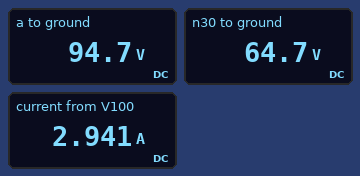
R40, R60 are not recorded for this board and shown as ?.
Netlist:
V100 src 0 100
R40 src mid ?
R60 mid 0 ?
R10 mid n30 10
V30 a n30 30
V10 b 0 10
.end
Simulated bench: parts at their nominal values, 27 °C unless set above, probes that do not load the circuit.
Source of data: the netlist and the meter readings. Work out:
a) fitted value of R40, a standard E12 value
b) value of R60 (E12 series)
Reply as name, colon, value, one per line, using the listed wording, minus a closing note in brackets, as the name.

fitted value of R40, a standard E12 value: 12 Ω
value of R60: 22 Ω
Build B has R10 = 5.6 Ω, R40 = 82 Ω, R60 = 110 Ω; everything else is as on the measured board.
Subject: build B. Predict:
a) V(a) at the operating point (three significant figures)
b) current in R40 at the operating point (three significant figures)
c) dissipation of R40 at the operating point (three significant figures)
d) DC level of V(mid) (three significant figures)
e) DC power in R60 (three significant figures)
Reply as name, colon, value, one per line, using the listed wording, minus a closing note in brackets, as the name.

V(a) at the operating point: 87.3 V
current in R40 at the operating point: 521 mA
dissipation of R40 at the operating point: 22.2 W
DC level of V(mid): 57.3 V
DC power in R60: 29.8 W
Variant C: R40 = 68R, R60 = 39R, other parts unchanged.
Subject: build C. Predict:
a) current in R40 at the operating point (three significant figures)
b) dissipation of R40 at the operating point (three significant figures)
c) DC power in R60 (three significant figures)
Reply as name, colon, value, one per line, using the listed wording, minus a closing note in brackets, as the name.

current in R40 at the operating point: 935 mA
dissipation of R40 at the operating point: 59.4 W
DC power in R60: 34.1 W
